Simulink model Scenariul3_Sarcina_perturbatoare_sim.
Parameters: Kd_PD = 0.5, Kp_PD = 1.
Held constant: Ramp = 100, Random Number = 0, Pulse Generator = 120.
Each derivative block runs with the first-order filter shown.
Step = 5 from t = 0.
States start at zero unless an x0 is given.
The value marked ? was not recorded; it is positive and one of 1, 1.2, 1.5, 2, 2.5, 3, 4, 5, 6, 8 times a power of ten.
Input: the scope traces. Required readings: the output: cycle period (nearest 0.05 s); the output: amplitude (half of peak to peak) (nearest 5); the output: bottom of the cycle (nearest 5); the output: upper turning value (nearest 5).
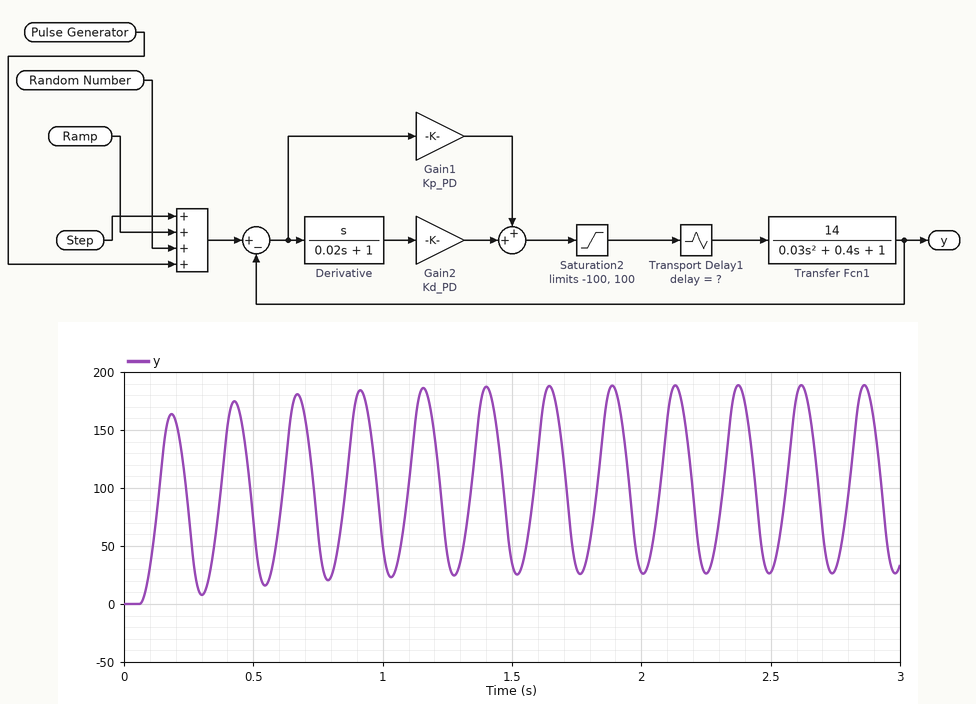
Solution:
0.25 s
80
25
190
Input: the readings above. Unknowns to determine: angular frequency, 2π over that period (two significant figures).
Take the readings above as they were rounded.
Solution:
25 rad/s
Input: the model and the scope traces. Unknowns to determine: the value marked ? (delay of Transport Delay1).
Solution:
0.06
